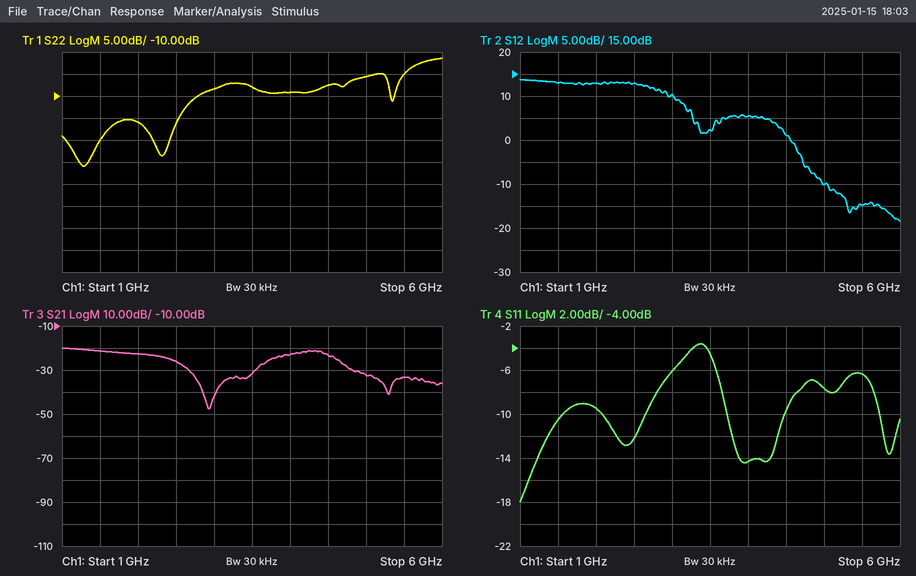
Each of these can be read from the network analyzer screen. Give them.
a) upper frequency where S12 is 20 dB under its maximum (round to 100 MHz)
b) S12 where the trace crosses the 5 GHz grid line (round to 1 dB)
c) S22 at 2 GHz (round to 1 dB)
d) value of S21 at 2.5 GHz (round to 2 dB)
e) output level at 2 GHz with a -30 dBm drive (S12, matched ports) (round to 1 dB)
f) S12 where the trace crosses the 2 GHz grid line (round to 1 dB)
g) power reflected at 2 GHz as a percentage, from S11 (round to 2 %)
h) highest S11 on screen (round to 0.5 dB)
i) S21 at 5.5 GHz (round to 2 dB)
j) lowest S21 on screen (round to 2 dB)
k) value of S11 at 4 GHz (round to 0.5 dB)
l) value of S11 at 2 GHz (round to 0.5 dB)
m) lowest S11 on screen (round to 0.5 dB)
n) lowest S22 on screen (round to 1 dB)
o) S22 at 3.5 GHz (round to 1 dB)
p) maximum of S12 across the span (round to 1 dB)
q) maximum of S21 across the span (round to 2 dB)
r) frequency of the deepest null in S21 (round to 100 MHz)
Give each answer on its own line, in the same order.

4.8 GHz
-10 dB
-16 dB
-26 dB
-17 dBm
13 dB
12 %
-3.5 dB
-34 dB
-48 dB
-14.5 dB
-9.5 dB
-18.0 dB
-26 dB
-8 dB
14 dB
-20 dB
2.9 GHz
